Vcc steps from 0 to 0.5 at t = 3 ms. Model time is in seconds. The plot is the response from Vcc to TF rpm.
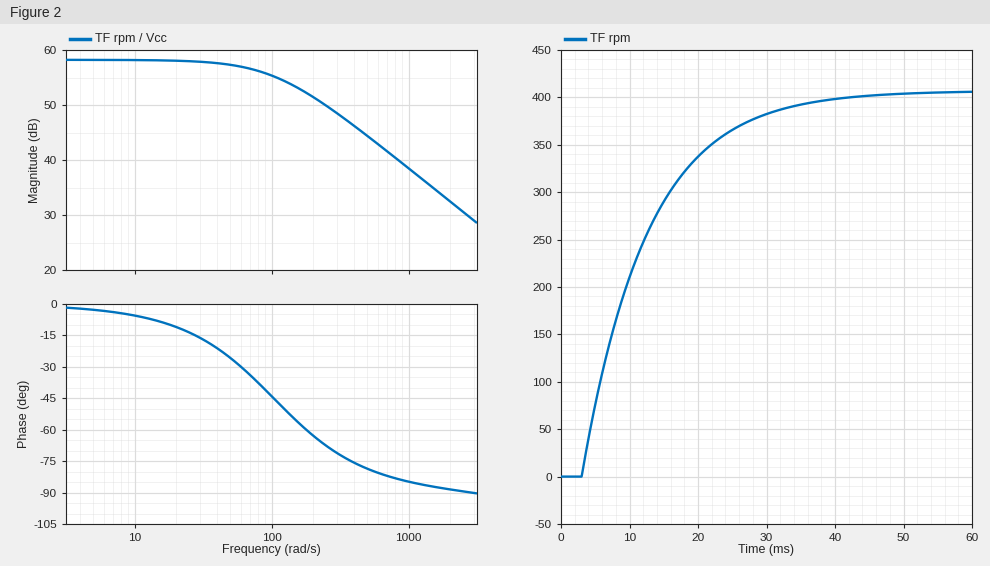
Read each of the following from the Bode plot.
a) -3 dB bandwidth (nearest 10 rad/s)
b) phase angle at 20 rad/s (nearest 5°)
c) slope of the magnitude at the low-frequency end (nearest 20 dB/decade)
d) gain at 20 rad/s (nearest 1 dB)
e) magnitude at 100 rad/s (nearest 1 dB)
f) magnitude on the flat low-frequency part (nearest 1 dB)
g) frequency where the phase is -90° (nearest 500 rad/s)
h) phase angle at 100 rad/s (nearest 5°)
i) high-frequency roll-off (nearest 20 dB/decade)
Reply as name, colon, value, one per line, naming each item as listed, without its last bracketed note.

-3 dB bandwidth: 100 rad/s
phase angle at 20 rad/s: -10°
slope of the magnitude at the low-frequency end: 0 dB/decade
gain at 20 rad/s: 58 dB
magnitude at 100 rad/s: 55 dB
magnitude on the flat low-frequency part: 58 dB
frequency where the phase is -90°: 3000 rad/s
phase angle at 100 rad/s: -45°
high-frequency roll-off: -20 dB/decade
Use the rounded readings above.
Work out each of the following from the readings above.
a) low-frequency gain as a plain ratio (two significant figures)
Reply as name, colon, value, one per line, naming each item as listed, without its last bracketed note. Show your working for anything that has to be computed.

low-frequency gain as a plain ratio: 10^(58 / 20) = 790
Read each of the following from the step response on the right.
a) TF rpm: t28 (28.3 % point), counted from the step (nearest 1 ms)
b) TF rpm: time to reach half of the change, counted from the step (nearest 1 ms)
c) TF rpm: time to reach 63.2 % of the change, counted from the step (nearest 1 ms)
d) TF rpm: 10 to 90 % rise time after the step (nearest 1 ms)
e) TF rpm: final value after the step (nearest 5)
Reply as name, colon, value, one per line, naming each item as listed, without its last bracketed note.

TF rpm: t28 (28.3 % point), counted from the step: 3 ms
TF rpm: time to reach half of the change, counted from the step: 7 ms
TF rpm: time to reach 63.2 % of the change, counted from the step: 10 ms
TF rpm: 10 to 90 % rise time after the step: 21 ms
TF rpm: final value after the step: 405
